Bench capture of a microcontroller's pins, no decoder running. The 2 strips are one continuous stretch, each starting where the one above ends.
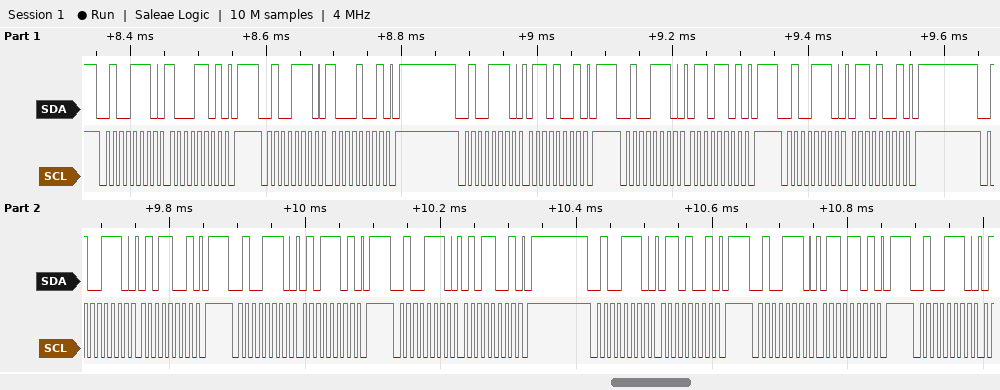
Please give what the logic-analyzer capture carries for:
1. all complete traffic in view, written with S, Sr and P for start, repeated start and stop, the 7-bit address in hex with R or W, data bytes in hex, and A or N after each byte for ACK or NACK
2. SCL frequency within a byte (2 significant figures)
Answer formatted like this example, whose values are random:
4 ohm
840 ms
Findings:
S 27W A 8D A P S 27W A 89 A P S 27W A 69 A P S 27W A 6D A P S 27W A 69 A P S 27W A 59 A P S 27W A 5D A P S 27W A 59 A P S 27W A 69 A P S 27W A 6D A P S 27W A
100 kHz
